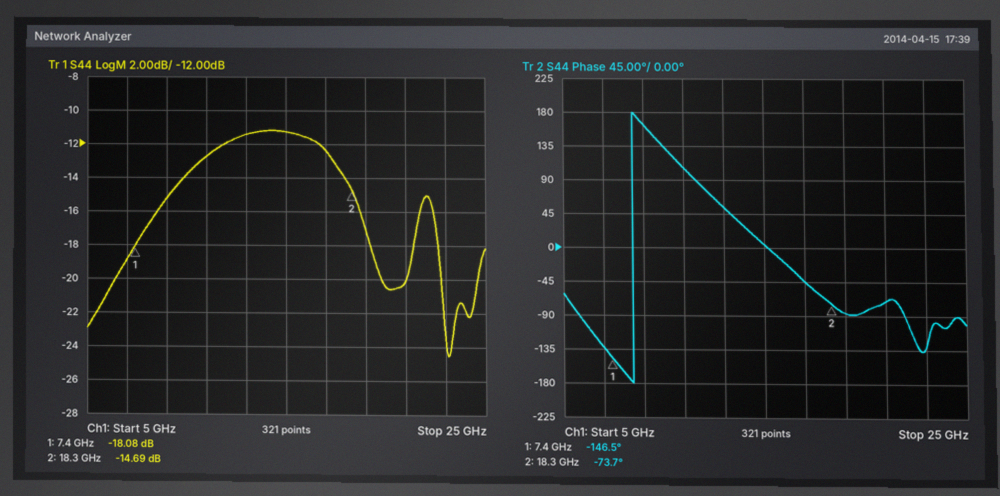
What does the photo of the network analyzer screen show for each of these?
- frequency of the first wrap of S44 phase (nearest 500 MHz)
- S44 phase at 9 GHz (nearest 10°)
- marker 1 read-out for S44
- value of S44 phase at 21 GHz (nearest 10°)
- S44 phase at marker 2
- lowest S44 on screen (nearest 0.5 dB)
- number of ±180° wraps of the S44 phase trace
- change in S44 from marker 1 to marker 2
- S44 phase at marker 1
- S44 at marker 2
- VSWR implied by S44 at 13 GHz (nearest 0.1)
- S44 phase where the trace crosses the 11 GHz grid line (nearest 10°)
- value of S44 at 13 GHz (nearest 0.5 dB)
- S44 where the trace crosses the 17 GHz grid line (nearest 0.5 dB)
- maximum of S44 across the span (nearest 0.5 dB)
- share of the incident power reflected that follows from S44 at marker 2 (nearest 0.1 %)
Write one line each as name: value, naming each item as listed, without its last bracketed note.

frequency of the first wrap of S44 phase: 8.5 GHz
S44 phase at 9 GHz: 160°
marker 1 read-out for S44: -18.08 dB
value of S44 phase at 21 GHz: -70°
S44 phase at marker 2: -73.7°
lowest S44 on screen: -24.5 dB
number of ±180° wraps of the S44 phase trace: 1
change in S44 from marker 1 to marker 2: 3.39 dB
S44 phase at marker 1: -146.5°
S44 at marker 2: -14.69 dB
VSWR implied by S44 at 13 GHz: 1.7
S44 phase where the trace crosses the 11 GHz grid line: 110°
value of S44 at 13 GHz: -11.5 dB
S44 where the trace crosses the 17 GHz grid line: -12.5 dB
maximum of S44 across the span: -11.0 dB
share of the incident power reflected that follows from S44 at marker 2: 3.4 %
